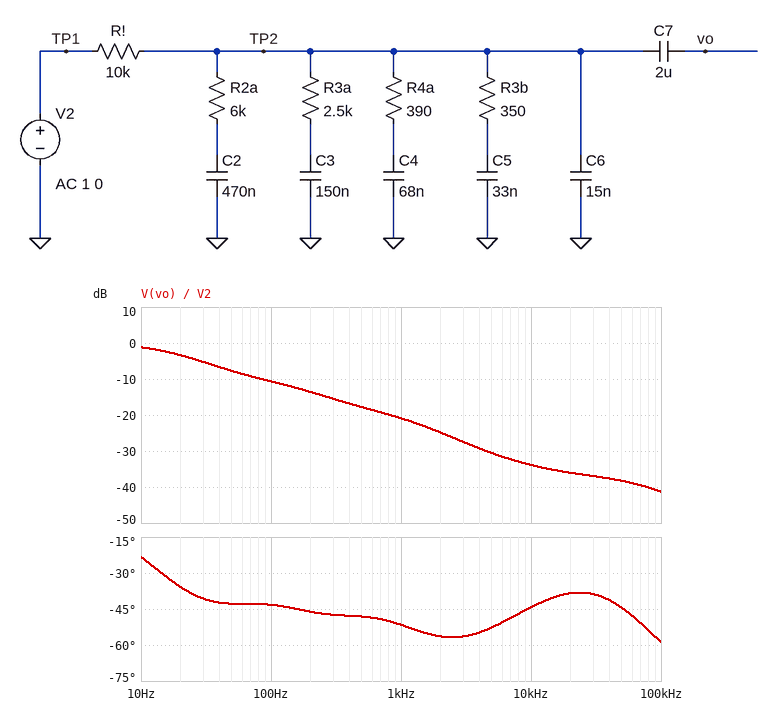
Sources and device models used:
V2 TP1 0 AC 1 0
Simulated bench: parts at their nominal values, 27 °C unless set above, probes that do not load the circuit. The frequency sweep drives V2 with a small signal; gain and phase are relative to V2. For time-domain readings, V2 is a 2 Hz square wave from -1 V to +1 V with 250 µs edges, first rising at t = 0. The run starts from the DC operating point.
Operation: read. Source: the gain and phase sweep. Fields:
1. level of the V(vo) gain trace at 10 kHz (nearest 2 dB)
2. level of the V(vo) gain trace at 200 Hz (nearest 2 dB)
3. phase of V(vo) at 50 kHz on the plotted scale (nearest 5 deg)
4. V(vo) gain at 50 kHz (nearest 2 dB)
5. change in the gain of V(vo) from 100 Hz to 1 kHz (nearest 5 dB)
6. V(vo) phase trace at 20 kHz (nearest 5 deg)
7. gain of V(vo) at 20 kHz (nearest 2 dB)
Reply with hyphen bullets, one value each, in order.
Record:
- -34 dB
- -14 dB
- -45 deg
- -38 dB
- -10 dB
- -40 deg
- -36 dB
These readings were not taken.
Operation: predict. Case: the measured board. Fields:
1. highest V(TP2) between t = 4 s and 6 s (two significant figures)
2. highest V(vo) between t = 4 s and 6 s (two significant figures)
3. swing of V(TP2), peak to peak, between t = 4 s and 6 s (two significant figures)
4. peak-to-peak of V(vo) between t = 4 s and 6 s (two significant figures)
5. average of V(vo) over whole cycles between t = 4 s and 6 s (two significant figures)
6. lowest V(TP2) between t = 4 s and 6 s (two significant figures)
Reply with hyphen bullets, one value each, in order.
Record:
- 1.0 V
- 2.0 V
- 2.0 V
- 2.0 V
- 1.0 V
- -1.0 V
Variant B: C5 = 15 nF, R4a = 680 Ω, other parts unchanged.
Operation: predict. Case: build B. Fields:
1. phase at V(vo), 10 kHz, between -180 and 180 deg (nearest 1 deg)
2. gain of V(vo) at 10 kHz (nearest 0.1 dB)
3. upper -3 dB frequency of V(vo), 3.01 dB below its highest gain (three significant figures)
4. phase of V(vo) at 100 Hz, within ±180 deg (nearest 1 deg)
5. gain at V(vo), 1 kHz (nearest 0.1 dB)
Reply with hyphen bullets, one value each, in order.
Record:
- -45 deg
- -30.1 dB
- 18.7 Hz
- -42 deg
- -20.3 dB
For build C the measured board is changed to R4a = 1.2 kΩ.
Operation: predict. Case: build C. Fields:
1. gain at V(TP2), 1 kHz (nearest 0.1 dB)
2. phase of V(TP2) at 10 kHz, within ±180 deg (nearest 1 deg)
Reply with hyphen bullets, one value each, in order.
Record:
- -21.0 dB
- -45 deg
